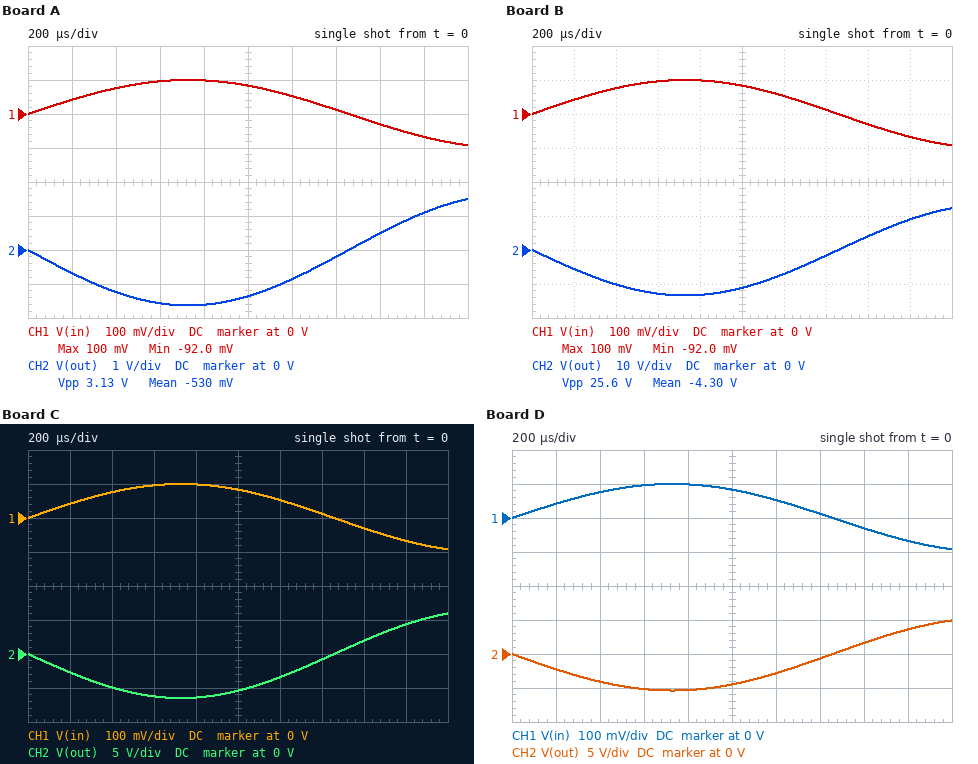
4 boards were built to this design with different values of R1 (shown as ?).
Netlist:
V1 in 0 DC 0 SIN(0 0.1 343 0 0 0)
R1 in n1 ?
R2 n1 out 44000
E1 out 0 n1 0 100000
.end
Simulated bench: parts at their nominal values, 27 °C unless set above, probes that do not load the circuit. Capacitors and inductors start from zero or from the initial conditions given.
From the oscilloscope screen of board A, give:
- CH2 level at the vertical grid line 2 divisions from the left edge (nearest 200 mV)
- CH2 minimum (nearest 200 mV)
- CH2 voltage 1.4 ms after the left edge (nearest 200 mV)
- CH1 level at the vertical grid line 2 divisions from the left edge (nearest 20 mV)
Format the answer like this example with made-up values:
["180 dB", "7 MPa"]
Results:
["-1.2 V", "-1.6 V", "-200 mV", "80 mV"]
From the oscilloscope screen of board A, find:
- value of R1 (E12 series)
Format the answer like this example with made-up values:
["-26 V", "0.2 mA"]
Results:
["2.7 kΩ"]
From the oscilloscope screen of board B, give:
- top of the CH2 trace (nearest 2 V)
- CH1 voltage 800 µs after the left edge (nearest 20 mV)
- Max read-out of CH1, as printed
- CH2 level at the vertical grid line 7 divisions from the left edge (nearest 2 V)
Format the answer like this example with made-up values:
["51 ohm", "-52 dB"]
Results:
["12 V", "100 mV", "100 mV", "-2 V"]
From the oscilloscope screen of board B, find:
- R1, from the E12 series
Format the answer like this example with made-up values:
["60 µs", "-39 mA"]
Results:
["330 Ω"]
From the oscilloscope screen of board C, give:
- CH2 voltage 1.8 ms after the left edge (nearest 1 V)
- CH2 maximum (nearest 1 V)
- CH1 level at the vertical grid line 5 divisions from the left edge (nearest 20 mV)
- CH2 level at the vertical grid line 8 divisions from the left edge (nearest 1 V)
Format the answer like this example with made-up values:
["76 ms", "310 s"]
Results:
["4 V", "6 V", "80 mV", "2 V"]
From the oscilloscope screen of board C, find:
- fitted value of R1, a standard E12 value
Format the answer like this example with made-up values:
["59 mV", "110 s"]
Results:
["680 Ω"]
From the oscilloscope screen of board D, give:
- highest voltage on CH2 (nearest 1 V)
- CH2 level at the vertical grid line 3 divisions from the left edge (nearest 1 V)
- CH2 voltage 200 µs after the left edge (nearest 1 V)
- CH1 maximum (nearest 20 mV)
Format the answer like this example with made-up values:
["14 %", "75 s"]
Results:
["5 V", "-5 V", "-2 V", "100 mV"]
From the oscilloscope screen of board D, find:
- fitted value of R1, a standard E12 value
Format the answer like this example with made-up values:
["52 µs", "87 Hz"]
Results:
["820 Ω"]
